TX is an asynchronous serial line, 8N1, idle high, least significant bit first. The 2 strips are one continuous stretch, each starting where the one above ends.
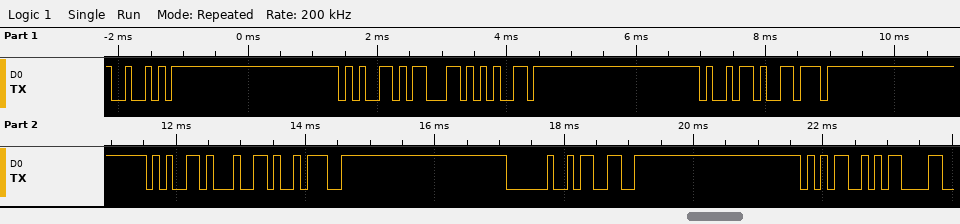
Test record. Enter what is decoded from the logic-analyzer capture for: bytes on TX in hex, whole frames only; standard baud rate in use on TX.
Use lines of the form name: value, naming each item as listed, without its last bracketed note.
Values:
bytes on TX in hex, whole frames only: 0x52 0x65 0x63 0x65 0x69 0x76 0x65 0x64 0x3A 0x20 0x33 0x35 0x0D
standard baud rate in use on TX: 9600 baud
